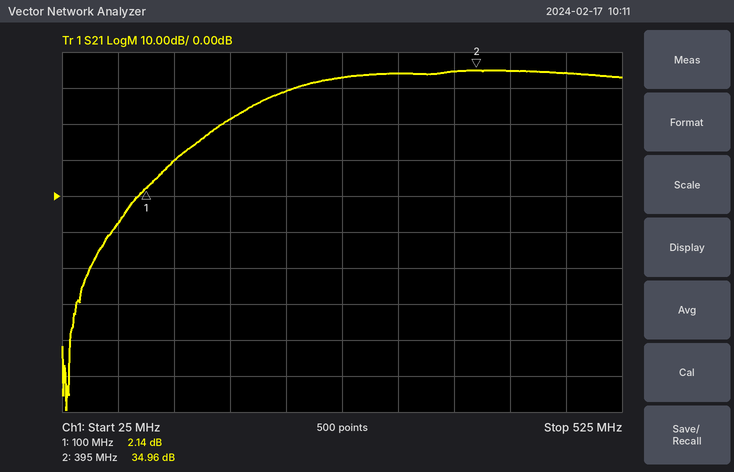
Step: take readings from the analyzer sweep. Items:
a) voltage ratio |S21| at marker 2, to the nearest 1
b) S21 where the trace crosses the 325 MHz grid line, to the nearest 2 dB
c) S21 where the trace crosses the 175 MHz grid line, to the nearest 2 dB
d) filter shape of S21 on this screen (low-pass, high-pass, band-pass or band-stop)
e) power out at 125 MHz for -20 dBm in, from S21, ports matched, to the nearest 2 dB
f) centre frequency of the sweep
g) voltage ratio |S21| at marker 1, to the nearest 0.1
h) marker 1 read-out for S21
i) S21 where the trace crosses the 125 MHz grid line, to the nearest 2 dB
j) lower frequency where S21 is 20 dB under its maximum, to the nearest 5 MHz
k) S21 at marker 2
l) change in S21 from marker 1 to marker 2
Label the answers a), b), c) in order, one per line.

a) 56
b) 34 dB
c) 22 dB
d) high-pass
e) -10 dBm
f) 275 MHz
g) 1.3
h) 2.14 dB
i) 10 dB
j) 145 MHz
k) 34.96 dB
l) 32.82 dB
